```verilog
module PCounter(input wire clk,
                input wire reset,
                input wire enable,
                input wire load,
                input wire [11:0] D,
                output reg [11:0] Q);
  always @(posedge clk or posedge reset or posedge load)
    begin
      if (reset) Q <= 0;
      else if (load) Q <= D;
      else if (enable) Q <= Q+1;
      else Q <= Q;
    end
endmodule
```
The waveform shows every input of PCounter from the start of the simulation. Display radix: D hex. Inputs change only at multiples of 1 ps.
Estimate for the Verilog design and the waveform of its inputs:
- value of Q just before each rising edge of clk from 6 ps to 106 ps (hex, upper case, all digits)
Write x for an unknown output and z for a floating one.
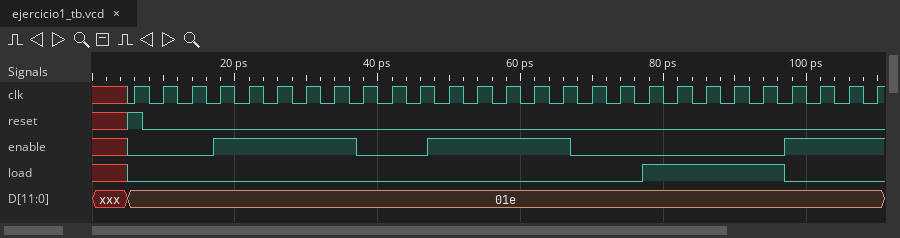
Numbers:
000, 000, 000, 000, 001, 002, 003, 004, 005, 005, 005, 005, 006, 007, 008, 009, 00A, 00A, 01E, 01E, 01E, 01E, 01E, 01E, 01F, 020
